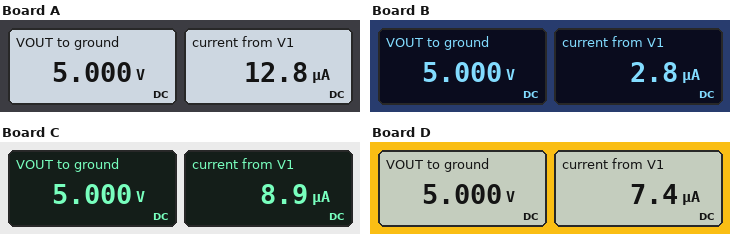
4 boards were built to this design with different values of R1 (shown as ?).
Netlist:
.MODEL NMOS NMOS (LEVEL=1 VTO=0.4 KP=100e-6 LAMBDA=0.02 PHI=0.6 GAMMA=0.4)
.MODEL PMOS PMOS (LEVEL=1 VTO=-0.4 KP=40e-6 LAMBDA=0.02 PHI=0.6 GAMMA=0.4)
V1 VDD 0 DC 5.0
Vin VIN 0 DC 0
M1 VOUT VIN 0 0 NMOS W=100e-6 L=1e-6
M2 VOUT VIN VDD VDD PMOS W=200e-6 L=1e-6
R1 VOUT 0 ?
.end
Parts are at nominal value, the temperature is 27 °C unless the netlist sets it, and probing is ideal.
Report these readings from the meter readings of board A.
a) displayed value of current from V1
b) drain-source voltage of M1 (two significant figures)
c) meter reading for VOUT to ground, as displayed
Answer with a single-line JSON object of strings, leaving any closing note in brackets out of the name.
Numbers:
{"displayed value of current from V1": "12.8 µA", "drain-source voltage of M1": "5.0 V", "meter reading for VOUT to ground, as displayed": "5.000 V"}
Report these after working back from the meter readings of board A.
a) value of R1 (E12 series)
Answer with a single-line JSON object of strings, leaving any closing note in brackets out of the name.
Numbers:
{"value of R1": "390 kΩ"}
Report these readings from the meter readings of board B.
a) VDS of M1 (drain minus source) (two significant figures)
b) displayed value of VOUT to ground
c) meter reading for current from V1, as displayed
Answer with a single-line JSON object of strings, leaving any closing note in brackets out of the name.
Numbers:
{"VDS of M1 (drain minus source)": "5.0 V", "displayed value of VOUT to ground": "5.000 V", "meter reading for current from V1, as displayed": "2.8 µA"}
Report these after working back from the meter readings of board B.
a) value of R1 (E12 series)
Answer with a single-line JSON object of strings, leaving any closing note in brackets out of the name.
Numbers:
{"value of R1": "1.8 MΩ"}
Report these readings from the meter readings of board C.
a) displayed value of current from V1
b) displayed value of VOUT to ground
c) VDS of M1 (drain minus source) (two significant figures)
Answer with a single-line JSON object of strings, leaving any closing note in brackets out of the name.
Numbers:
{"displayed value of current from V1": "8.9 µA", "displayed value of VOUT to ground": "5.000 V", "VDS of M1 (drain minus source)": "5.0 V"}
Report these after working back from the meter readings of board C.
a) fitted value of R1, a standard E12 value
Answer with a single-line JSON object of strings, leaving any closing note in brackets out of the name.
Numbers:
{"fitted value of R1, a standard E12 value": "560 kΩ"}
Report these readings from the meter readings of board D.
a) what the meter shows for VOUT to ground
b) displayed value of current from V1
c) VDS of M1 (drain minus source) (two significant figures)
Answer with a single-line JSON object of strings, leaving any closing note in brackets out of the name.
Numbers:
{"what the meter shows for VOUT to ground": "5.000 V", "displayed value of current from V1": "7.4 µA", "VDS of M1 (drain minus source)": "5.0 V"}
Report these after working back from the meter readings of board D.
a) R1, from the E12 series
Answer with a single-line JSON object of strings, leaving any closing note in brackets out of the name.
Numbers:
{"R1, from the E12 series": "680 kΩ"}
